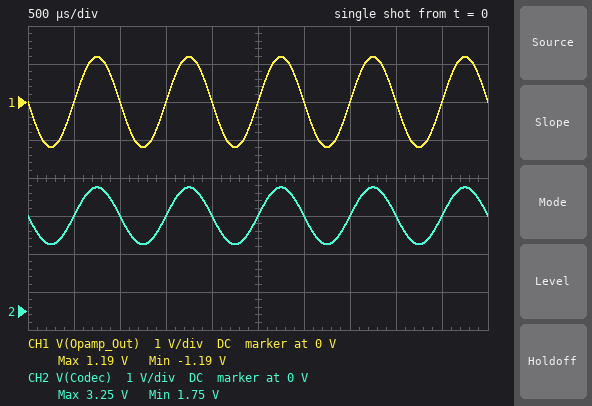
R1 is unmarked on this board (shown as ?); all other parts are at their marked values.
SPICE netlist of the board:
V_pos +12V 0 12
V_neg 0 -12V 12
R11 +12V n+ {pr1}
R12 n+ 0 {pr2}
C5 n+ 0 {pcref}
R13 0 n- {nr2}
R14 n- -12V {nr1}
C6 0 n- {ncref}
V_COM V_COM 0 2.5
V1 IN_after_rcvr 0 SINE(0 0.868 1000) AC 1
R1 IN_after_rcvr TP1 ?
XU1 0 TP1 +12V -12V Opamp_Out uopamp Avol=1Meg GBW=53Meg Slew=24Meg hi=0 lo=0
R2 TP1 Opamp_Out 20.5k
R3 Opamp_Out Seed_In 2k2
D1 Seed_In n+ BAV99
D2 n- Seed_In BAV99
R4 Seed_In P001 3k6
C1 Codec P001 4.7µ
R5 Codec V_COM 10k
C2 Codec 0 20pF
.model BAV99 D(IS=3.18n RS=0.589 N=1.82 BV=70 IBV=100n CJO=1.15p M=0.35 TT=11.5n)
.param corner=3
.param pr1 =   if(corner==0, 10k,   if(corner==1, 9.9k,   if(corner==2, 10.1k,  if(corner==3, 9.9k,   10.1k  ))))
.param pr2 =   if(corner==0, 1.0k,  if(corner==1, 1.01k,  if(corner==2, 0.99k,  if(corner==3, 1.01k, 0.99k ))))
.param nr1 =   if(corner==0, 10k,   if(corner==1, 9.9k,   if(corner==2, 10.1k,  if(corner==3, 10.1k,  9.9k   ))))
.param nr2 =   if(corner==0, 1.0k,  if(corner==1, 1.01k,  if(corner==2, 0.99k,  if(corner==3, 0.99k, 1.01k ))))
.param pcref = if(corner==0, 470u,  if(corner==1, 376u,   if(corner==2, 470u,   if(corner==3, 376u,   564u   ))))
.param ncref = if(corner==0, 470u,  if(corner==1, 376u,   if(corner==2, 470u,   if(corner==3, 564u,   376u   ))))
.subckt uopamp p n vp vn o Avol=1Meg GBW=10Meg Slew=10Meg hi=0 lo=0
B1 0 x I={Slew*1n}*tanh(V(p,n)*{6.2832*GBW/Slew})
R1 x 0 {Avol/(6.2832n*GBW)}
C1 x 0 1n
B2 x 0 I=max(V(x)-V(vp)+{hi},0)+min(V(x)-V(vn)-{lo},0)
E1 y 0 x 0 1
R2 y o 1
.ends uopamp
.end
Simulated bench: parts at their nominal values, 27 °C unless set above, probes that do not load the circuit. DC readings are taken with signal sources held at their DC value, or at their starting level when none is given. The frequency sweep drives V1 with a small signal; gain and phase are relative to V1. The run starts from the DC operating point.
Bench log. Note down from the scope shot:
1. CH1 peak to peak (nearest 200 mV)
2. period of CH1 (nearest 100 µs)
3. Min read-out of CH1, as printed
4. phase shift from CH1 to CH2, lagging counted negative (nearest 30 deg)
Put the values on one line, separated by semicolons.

2.4 V; 1.0 ms; -1.19 V; 0 deg
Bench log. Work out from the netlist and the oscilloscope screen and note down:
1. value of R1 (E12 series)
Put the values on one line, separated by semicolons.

15 kΩ
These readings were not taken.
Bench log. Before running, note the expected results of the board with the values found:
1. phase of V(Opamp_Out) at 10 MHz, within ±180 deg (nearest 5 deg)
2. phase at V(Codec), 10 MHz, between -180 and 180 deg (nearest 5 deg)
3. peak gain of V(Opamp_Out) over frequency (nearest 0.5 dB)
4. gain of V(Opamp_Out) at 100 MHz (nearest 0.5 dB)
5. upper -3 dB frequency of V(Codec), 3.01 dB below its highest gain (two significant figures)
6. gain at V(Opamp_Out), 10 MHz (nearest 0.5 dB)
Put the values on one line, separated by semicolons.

155 deg; 70 deg; 2.5 dB; -10.5 dB; 2.1 MHz; 2.0 dB
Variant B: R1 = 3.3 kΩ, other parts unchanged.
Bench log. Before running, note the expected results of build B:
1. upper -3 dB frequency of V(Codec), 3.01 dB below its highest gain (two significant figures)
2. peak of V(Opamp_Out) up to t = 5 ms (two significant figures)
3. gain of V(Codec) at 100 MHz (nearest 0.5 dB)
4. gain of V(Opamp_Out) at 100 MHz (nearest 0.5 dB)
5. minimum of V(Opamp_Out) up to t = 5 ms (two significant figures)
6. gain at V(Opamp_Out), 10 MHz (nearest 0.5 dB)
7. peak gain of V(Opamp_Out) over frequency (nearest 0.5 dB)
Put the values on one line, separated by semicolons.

2.0 MHz; 5.4 V; -49.5 dB; -7.0 dB; -5.4 V; 11.5 dB; 16.0 dB
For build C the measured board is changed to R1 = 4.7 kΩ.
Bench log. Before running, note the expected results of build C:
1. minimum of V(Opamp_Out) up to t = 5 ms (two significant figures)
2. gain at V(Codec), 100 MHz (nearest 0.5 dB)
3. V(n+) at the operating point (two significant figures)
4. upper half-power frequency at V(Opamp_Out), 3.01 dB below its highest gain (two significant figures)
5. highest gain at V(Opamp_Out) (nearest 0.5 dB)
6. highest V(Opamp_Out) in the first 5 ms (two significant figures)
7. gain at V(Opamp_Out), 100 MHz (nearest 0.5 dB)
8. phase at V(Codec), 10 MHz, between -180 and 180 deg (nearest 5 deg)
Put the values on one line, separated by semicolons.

-3.8 V; -50.0 dB; 1.1 V; 9.9 MHz; 13.0 dB; 3.8 V; -7.5 dB; 50 deg
